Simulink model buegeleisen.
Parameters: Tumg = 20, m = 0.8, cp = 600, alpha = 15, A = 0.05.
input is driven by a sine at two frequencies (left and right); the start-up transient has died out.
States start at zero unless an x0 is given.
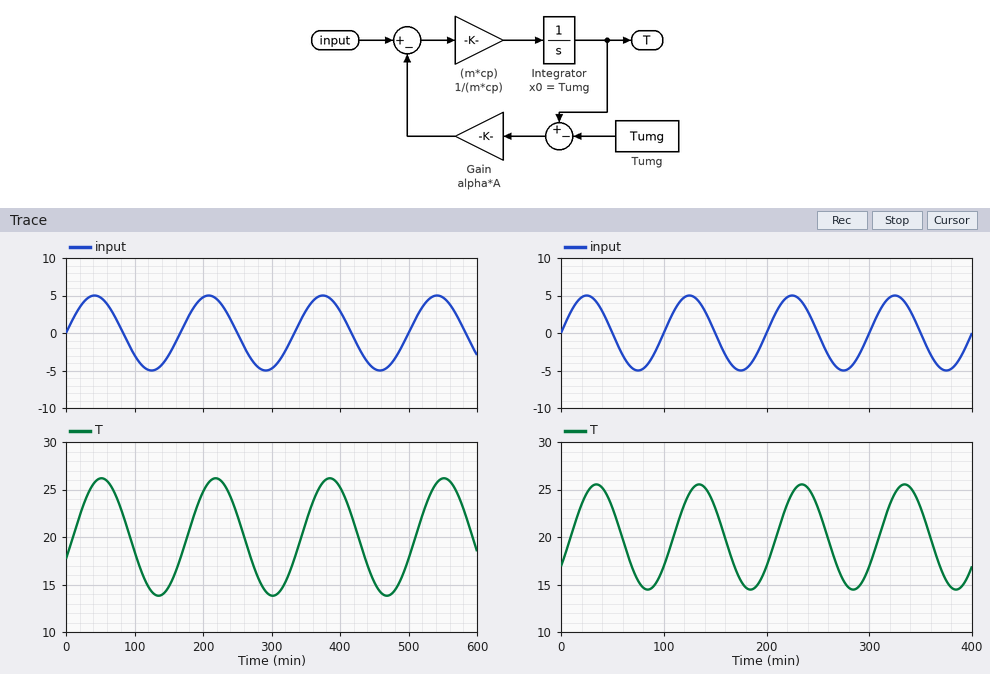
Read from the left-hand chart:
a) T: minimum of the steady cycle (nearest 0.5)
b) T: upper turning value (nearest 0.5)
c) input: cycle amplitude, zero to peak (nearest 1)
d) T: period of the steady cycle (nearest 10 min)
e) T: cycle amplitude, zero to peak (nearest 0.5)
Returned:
14.0
26.0
5
170 min
6.0
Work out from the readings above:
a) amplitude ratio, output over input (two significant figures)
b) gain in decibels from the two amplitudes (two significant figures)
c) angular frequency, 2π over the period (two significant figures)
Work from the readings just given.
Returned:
1.2
1.6 dB
0.037 rad/min
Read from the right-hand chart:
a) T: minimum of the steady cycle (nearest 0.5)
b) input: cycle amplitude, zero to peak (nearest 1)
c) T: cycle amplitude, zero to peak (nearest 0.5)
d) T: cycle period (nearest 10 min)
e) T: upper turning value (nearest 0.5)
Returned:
14.5
5
5.5
100 min
25.5
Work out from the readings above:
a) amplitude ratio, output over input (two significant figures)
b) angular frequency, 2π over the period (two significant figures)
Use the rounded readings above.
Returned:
1.1
0.063 rad/min
